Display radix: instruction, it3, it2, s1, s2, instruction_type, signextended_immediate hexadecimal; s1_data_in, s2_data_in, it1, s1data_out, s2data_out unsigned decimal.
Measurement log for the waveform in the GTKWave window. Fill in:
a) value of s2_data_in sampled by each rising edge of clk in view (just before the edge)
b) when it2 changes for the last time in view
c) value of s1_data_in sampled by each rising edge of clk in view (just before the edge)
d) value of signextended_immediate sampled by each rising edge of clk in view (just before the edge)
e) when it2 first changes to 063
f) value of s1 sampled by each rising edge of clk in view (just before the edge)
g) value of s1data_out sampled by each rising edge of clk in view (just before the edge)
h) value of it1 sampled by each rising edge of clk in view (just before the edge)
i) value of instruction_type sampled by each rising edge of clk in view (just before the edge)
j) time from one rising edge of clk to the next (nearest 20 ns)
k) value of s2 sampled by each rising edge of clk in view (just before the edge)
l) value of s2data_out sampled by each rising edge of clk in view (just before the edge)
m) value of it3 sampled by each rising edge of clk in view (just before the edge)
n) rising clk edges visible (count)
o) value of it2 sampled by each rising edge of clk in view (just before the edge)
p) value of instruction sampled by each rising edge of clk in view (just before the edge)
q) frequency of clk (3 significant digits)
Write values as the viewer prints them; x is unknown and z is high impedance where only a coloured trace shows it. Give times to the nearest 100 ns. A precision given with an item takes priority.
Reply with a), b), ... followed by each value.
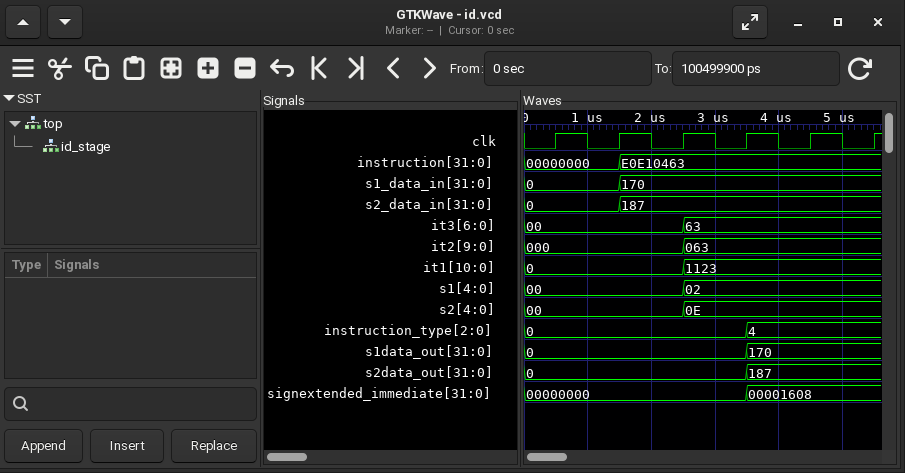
a) 0, 0, 187, 187, 187, 187
b) 2500 ns
c) 0, 0, 170, 170, 170, 170
d) 00000000, 00000000, 00000000, 00000000, 00001608, 00001608
e) 2500 ns
f) 00, 00, 00, 02, 02, 02
g) 0, 0, 0, 0, 170, 170
h) 0, 0, 0, 1123, 1123, 1123
i) 0, 0, 0, 0, 4, 4
j) 1000 ns
k) 00, 00, 00, 0E, 0E, 0E
l) 0, 0, 0, 0, 187, 187
m) 00, 00, 00, 63, 63, 63
n) 6
o) 000, 000, 000, 063, 063, 063
p) 00000000, 00000000, E0E10463, E0E10463, E0E10463, E0E10463
q) 1.00 MHz
